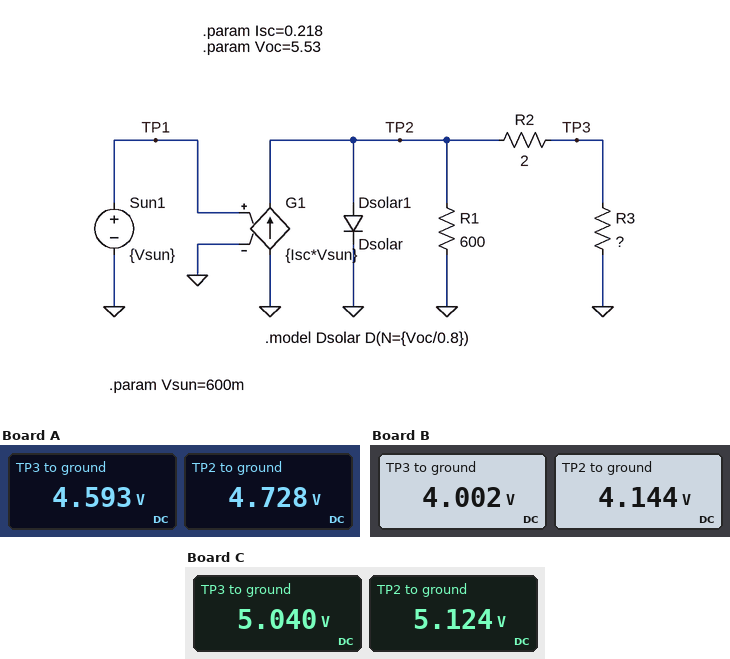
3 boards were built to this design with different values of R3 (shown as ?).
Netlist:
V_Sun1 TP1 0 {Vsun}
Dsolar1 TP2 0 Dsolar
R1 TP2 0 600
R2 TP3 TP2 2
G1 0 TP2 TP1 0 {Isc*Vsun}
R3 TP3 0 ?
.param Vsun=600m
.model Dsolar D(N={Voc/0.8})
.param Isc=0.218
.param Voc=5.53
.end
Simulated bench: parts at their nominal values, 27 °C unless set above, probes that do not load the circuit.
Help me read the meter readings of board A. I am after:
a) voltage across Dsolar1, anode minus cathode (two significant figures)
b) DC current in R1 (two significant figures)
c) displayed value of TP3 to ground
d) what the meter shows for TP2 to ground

4.7 V
7.9 mA
4.593 V
4.728 V
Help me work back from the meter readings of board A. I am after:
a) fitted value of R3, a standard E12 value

68 Ω
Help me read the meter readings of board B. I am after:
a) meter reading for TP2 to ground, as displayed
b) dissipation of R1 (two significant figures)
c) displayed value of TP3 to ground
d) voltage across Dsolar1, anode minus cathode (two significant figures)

4.144 V
29 mW
4.002 V
4.1 V
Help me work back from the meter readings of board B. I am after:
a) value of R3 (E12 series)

56 Ω
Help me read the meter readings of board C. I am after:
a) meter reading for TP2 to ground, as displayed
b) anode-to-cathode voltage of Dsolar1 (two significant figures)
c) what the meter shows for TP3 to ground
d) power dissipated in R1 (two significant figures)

5.124 V
5.1 V
5.040 V
44 mW
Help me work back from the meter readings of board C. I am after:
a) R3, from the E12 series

120 Ω
